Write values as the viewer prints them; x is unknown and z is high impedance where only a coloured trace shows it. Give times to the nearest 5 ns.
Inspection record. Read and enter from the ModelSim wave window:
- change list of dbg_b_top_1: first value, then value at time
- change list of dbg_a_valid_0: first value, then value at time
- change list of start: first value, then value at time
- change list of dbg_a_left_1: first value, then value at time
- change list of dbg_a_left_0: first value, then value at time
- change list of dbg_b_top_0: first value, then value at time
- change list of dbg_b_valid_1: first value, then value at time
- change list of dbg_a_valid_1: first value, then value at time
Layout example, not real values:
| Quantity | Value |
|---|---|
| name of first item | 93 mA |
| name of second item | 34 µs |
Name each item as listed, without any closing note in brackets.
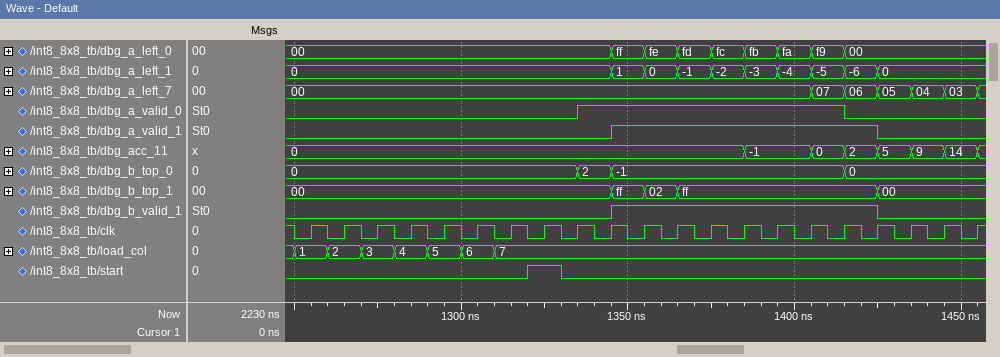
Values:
| Quantity | Value |
|---|---|
| change list of dbg_b_top_1: first value, then value at time | 00, ff at 1345 ns, 02 at 1355 ns, ff at 1365 ns, 00 at 1425 ns |
| change list of dbg_a_valid_0: first value, then value at time | 0, 1 at 1335 ns, 0 at 1415 ns |
| change list of start: first value, then value at time | 0, 1 at 1320 ns, 0 at 1330 ns |
| change list of dbg_a_left_1: first value, then value at time | 0, 1 at 1345 ns, 0 at 1355 ns, -1 at 1365 ns, -2 at 1375 ns, -3 at 1385 ns, -4 at 1395 ns, -5 at 1405 ns, -6 at 1415 ns, 0 at 1425 ns |
| change list of dbg_a_left_0: first value, then value at time | 00, ff at 1345 ns, fe at 1355 ns, fd at 1365 ns, fc at 1375 ns, fb at 1385 ns, fa at 1395 ns, f9 at 1405 ns, 00 at 1415 ns |
| change list of dbg_b_top_0: first value, then value at time | 0, 2 at 1335 ns, -1 at 1345 ns, 0 at 1415 ns |
| change list of dbg_b_valid_1: first value, then value at time | 0, 1 at 1345 ns, 0 at 1425 ns |
| change list of dbg_a_valid_1: first value, then value at time | 0, 1 at 1345 ns, 0 at 1425 ns |
